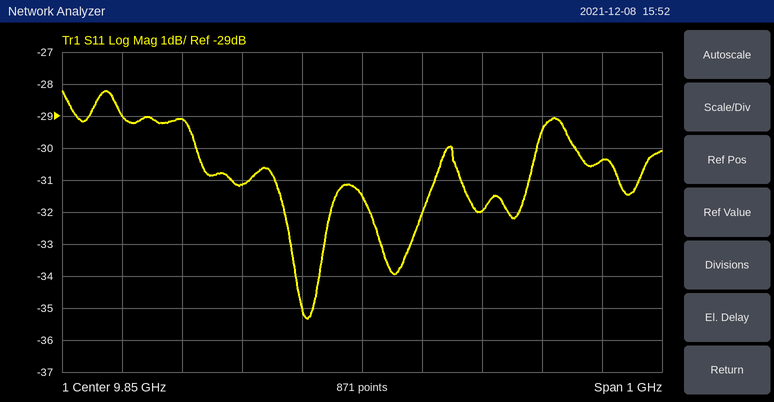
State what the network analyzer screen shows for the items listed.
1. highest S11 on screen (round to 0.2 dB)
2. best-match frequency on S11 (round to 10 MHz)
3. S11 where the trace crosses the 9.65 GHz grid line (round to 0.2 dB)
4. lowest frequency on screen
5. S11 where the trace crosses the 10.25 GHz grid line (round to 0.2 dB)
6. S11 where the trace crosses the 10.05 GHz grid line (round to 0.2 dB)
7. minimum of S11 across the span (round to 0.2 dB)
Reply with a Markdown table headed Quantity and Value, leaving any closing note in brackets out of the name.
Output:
| Quantity | Value |
|---|---|
| highest S11 on screen | -28.2 dB |
| best-match frequency on S11 | 9.76 GHz |
| S11 where the trace crosses the 9.65 GHz grid line | -31.2 dB |
| lowest frequency on screen | 9.35 GHz |
| S11 where the trace crosses the 10.25 GHz grid line | -30.4 dB |
| S11 where the trace crosses the 10.05 GHz grid line | -32.0 dB |
| minimum of S11 across the span | -35.4 dB |
